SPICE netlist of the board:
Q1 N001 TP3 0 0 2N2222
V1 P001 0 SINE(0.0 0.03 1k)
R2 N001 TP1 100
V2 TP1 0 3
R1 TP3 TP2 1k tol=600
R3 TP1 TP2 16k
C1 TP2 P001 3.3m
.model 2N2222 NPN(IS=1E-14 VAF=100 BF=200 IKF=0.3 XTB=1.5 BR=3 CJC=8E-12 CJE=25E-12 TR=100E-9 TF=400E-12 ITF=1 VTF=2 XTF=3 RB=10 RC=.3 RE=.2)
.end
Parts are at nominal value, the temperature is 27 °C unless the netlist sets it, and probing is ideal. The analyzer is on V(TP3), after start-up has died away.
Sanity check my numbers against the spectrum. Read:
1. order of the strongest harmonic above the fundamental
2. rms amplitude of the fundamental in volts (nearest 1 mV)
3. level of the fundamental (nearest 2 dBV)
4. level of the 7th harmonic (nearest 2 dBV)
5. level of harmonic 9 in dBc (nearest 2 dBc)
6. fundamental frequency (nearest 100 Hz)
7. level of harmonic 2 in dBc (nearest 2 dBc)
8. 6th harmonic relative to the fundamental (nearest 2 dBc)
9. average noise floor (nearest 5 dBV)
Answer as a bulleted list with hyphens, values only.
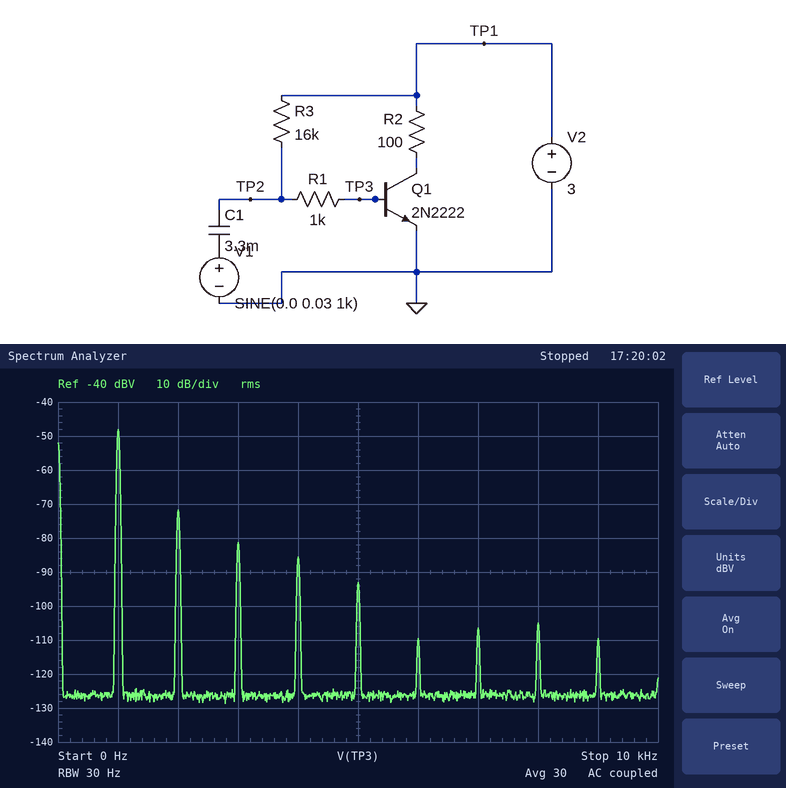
- 2
- 4 mV
- -48 dBV
- -106 dBV
- -62 dBc
- 1.0 kHz
- -24 dBc
- -62 dBc
- -125 dBV
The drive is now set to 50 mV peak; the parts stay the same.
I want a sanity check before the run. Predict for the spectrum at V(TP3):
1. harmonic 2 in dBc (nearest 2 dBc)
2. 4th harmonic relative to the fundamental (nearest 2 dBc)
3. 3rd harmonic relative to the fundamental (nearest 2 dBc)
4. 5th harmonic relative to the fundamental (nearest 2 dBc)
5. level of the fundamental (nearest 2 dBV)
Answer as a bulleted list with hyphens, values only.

- -16 dBc
- -40 dBc
- -26 dBc
- -40 dBc
- -44 dBV
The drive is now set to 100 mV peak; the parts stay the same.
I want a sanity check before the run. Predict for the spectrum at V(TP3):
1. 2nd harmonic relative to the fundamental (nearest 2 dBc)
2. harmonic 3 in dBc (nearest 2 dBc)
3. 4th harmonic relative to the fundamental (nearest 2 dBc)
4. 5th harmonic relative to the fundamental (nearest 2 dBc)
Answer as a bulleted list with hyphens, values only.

- -10 dBc
- -36 dBc
- -34 dBc
- -34 dBc
